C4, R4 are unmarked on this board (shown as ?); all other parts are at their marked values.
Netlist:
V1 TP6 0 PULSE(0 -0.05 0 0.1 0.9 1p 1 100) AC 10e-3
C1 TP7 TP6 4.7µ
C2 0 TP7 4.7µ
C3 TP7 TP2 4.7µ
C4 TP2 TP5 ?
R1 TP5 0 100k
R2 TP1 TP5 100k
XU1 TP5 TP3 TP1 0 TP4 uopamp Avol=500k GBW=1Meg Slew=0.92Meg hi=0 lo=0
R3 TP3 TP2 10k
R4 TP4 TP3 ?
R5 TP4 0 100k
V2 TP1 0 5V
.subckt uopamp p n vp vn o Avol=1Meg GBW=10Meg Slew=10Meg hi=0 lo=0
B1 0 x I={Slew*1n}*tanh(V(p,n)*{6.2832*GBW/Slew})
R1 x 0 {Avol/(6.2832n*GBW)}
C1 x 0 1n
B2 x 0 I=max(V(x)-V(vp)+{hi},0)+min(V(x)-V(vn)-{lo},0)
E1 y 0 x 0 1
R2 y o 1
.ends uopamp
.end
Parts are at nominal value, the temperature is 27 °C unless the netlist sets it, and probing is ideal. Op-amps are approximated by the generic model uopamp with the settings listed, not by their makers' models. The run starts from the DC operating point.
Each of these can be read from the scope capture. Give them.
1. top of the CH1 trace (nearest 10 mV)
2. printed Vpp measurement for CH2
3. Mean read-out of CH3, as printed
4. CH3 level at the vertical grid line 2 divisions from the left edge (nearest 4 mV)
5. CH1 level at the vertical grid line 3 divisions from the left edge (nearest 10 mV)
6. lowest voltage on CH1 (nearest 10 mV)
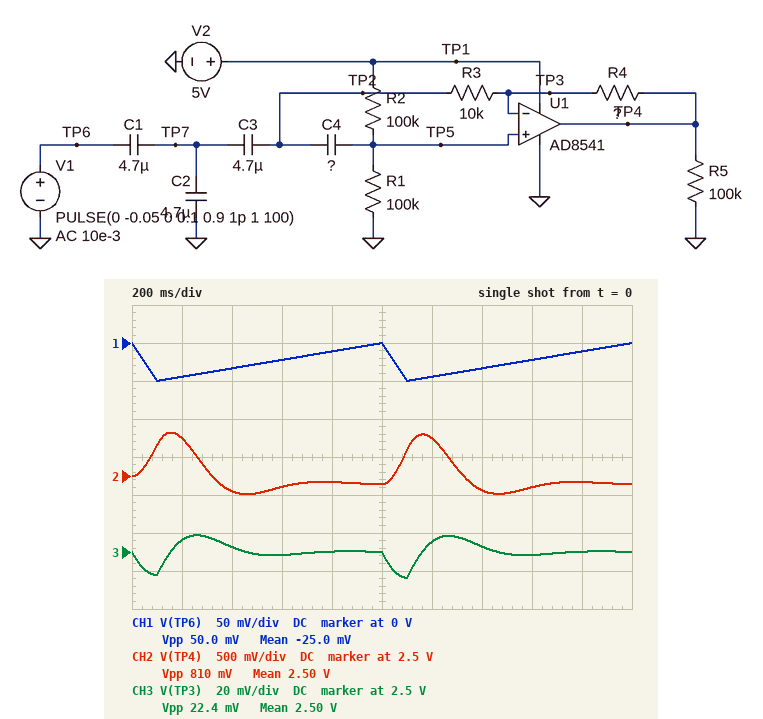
0 V
810 mV
2.50 V
2.504 V
-20 mV
-50 mV
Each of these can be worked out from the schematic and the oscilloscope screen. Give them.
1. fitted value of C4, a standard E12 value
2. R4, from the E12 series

4.7 µF
1.2 MΩ
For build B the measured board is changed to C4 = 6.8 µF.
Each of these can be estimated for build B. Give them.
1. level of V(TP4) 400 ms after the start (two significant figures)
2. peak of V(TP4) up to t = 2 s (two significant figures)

2.4 V
3.0 V
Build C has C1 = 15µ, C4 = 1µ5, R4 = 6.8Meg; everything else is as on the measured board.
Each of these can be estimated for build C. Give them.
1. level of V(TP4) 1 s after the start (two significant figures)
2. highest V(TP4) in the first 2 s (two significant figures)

1.4 V
5.0 V
